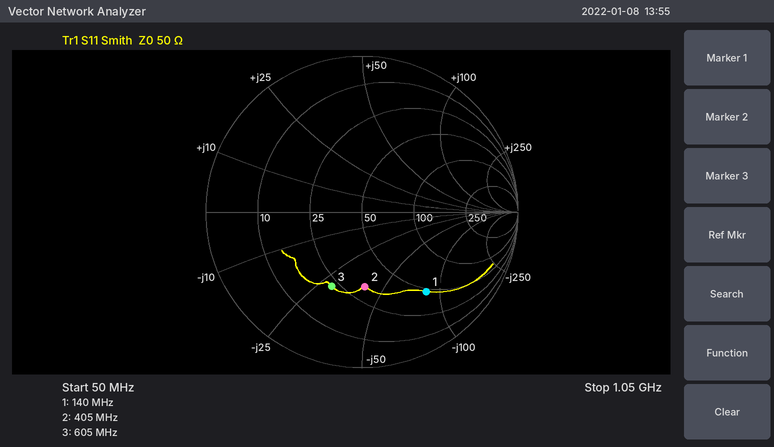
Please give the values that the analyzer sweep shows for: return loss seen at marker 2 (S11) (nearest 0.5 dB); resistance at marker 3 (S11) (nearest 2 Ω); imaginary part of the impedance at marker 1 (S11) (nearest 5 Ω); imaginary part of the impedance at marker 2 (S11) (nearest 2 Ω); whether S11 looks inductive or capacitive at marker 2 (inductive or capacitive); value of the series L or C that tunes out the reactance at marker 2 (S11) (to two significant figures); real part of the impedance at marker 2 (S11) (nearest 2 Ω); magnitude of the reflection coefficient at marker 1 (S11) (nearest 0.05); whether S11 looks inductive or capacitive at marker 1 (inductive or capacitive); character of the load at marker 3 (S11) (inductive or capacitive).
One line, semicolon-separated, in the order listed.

6.5 dB; 22 Ω; -85 Ω; -40 Ω; capacitive; 16 nH; 32 Ω; 0.65; capacitive; capacitive
